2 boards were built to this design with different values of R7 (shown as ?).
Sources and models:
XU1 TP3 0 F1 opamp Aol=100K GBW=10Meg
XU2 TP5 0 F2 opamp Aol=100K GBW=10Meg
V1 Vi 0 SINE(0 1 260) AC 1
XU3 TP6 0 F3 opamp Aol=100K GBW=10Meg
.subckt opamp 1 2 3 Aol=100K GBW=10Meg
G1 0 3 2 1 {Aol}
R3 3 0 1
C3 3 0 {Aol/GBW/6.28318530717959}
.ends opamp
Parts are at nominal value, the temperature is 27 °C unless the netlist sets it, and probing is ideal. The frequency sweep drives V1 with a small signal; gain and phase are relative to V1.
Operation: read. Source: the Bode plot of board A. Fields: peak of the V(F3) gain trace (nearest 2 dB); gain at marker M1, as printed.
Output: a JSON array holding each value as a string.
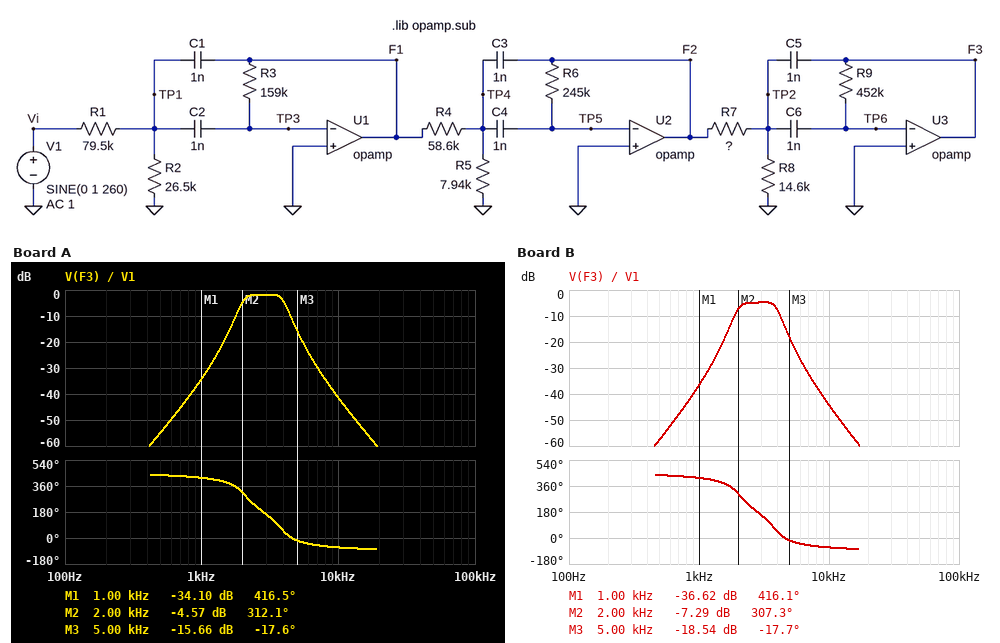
["-2 dB", "-34.10 dB"]
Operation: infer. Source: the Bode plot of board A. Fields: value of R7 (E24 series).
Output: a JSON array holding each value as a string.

["130 kΩ"]
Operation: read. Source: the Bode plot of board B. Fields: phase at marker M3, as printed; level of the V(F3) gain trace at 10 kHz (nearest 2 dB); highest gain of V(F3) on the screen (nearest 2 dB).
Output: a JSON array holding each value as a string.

["-17.7 deg", "-44 dB", "-4 dB"]
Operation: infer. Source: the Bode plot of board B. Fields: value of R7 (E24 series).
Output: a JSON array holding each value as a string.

["180 kΩ"]
